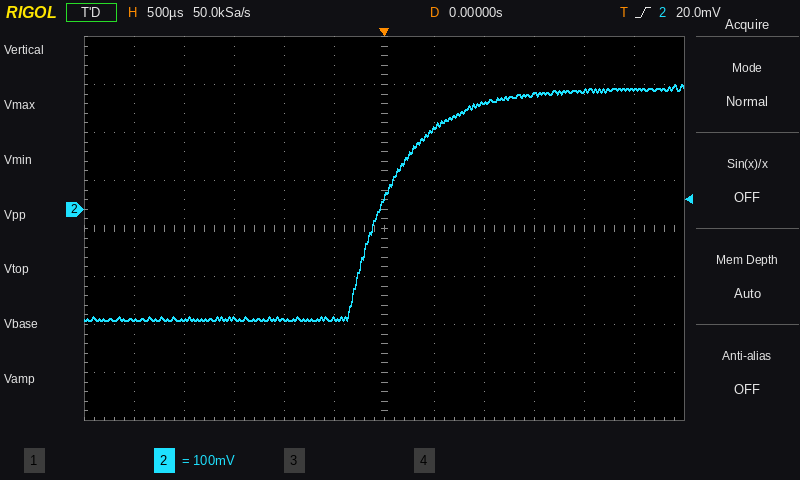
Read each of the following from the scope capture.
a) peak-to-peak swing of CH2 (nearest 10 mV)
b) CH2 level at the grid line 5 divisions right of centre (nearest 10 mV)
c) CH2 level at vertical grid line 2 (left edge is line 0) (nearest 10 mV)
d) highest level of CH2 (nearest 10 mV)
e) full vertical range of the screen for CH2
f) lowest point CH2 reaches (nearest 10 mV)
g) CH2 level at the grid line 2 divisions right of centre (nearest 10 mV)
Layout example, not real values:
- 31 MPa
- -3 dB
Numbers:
- 490 mV
- 250 mV
- -230 mV
- 260 mV
- 800 mV
- -230 mV
- 220 mV
